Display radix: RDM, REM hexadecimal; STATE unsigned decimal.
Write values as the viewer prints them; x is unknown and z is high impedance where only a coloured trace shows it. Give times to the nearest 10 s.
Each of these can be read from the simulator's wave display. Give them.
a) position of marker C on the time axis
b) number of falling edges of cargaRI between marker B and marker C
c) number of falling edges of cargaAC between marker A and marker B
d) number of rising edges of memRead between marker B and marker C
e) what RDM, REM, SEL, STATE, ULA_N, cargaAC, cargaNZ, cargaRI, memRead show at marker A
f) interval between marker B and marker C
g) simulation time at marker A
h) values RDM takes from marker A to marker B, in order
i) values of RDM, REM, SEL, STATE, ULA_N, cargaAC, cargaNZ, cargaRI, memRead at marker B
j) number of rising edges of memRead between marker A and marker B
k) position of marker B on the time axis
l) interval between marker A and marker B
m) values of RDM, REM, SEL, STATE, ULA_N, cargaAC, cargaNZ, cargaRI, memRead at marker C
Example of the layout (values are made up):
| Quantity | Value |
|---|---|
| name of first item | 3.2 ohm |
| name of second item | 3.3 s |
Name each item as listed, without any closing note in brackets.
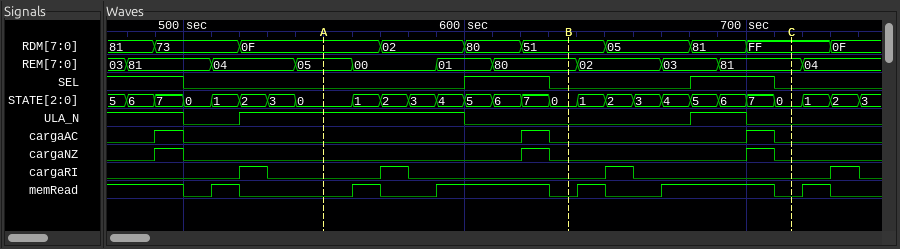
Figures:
| Quantity | Value |
|---|---|
| position of marker C on the time axis | 720 s |
| number of falling edges of cargaRI between marker B and marker C | 1 |
| number of falling edges of cargaAC between marker A and marker B | 1 |
| number of rising edges of memRead between marker B and marker C | 2 |
| what RDM, REM, SEL, STATE, ULA_N, cargaAC, cargaNZ, cargaRI, memRead show at marker A | RDM=0F, REM=05, SEL=0, STATE=0, ULA_N=1, cargaAC=0, cargaNZ=0, cargaRI=0, memRead=0 |
| interval between marker B and marker C | 80 s |
| simulation time at marker A | 550 s |
| values RDM takes from marker A to marker B, in order | 0F, 02, 80, 51 |
| values of RDM, REM, SEL, STATE, ULA_N, cargaAC, cargaNZ, cargaRI, memRead at marker B | RDM=51, REM=80, SEL=0, STATE=0, ULA_N=0, cargaAC=0, cargaNZ=0, cargaRI=0, memRead=0 |
| number of rising edges of memRead between marker A and marker B | 2 |
| position of marker B on the time axis | 640 s |
| interval between marker A and marker B | 90 s |
| values of RDM, REM, SEL, STATE, ULA_N, cargaAC, cargaNZ, cargaRI, memRead at marker C | RDM=FF, REM=81, SEL=0, STATE=0, ULA_N=0, cargaAC=0, cargaNZ=0, cargaRI=0, memRead=0 |
